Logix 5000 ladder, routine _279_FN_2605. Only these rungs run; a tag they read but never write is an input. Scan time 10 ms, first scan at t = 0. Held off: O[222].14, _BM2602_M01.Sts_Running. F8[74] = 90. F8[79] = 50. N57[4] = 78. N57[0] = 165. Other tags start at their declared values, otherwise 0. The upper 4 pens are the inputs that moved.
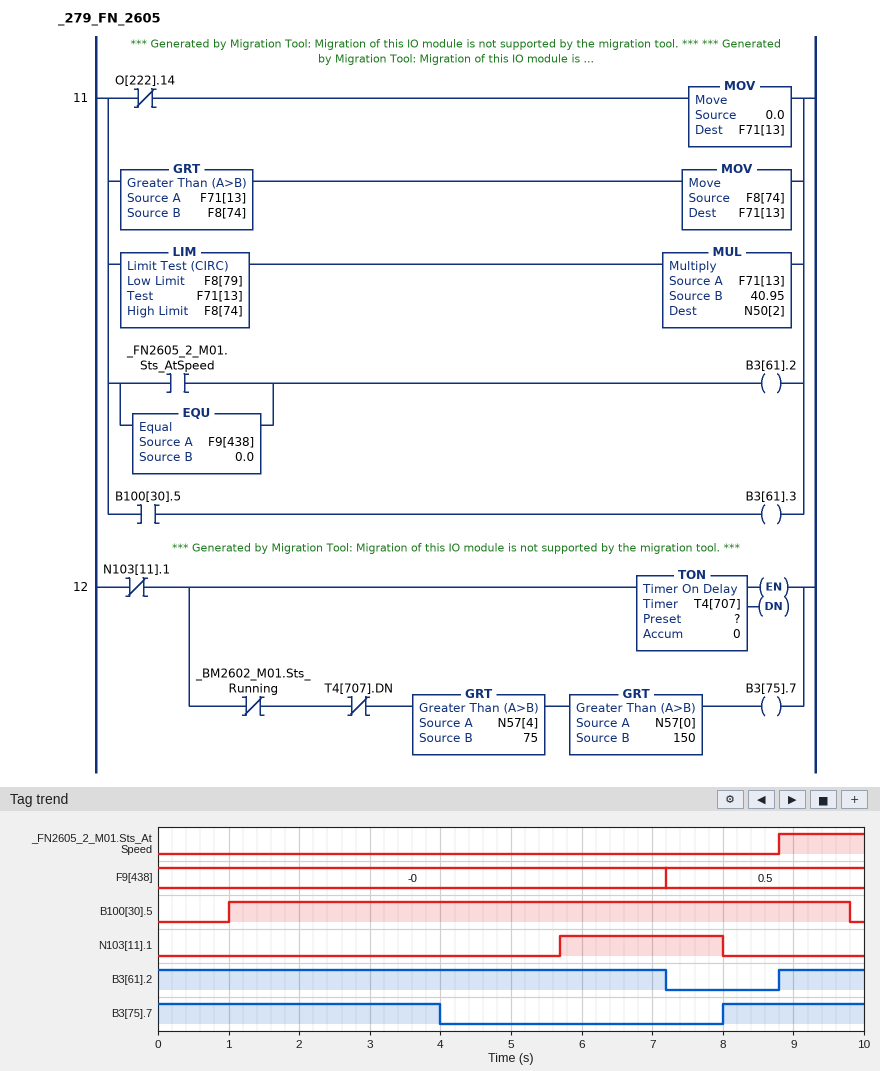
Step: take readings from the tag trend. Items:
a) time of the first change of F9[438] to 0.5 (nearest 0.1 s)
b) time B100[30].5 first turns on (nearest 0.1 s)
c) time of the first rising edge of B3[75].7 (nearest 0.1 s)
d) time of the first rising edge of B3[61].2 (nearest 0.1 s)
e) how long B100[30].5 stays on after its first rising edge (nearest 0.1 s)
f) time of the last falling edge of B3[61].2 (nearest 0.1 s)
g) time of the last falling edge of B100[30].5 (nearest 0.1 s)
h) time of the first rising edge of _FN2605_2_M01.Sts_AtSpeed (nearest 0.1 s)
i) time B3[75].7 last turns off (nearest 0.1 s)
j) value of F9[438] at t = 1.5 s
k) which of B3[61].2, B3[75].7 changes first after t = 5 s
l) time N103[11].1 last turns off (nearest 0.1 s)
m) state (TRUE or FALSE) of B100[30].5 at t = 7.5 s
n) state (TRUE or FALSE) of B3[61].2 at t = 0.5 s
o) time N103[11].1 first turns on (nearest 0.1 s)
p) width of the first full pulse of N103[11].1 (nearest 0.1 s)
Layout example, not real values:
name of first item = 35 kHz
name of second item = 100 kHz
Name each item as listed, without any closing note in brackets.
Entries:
time of the first change of F9[438] to 0.5 = 7.2 s
time B100[30].5 first turns on = 1.0 s
time of the first rising edge of B3[75].7 = 8.0 s
time of the first rising edge of B3[61].2 = 8.8 s
how long B100[30].5 stays on after its first rising edge = 8.8 s
time of the last falling edge of B3[61].2 = 7.2 s
time of the last falling edge of B100[30].5 = 9.8 s
time of the first rising edge of _FN2605_2_M01.Sts_AtSpeed = 8.8 s
time B3[75].7 last turns off = 4.0 s
value of F9[438] at t = 1.5 s = -0
which of B3[61].2, B3[75].7 changes first after t = 5 s = B3[61].2
time N103[11].1 last turns off = 8.0 s
state (TRUE or FALSE) of B100[30].5 at t = 7.5 s = TRUE
state (TRUE or FALSE) of B3[61].2 at t = 0.5 s = TRUE
time N103[11].1 first turns on = 5.7 s
width of the first full pulse of N103[11].1 = 2.3 s
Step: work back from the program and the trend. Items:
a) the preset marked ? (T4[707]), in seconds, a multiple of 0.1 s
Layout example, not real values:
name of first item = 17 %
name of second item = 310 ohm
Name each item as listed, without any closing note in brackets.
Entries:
the preset marked ? (T4[707]), in seconds, a multiple of 0.1 s = 4.0 s
